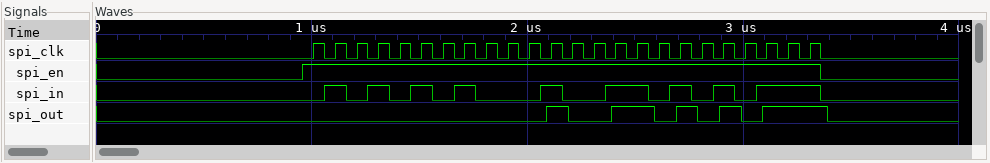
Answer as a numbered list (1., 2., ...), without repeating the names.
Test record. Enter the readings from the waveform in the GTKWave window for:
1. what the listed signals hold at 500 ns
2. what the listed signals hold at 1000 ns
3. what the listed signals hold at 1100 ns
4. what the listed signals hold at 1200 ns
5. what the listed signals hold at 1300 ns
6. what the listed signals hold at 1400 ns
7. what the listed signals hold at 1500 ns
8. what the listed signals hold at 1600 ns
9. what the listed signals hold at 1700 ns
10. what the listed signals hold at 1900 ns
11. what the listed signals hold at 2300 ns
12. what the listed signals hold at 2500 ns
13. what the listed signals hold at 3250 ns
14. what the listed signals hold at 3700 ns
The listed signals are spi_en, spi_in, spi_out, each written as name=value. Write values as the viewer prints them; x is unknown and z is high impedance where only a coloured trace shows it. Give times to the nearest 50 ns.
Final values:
1. spi_en=0, spi_in=0, spi_out=0
2. spi_en=1, spi_in=0, spi_out=0
3. spi_en=1, spi_in=1, spi_out=0
4. spi_en=1, spi_in=0, spi_out=0
5. spi_en=1, spi_in=1, spi_out=0
6. spi_en=1, spi_in=0, spi_out=0
7. spi_en=1, spi_in=1, spi_out=0
8. spi_en=1, spi_in=0, spi_out=0
9. spi_en=1, spi_in=1, spi_out=0
10. spi_en=1, spi_in=0, spi_out=0
11. spi_en=1, spi_in=0, spi_out=0
12. spi_en=1, spi_in=1, spi_out=1
13. spi_en=1, spi_in=1, spi_out=1
14. spi_en=0, spi_in=0, spi_out=0
